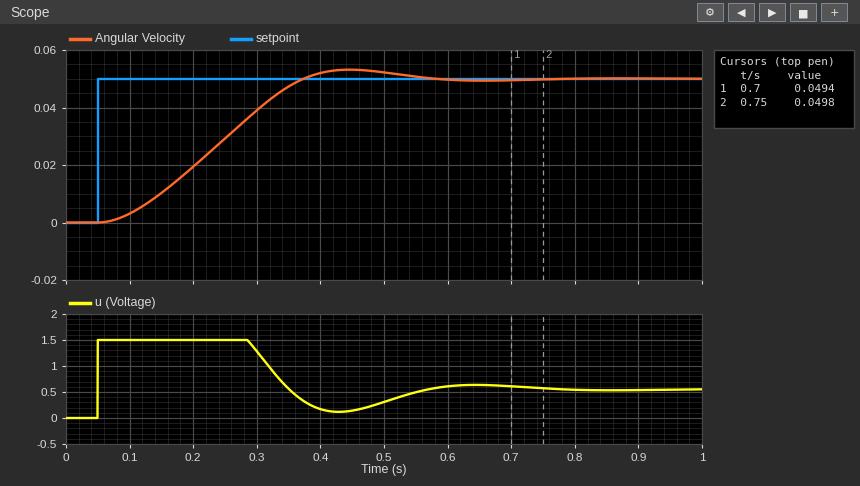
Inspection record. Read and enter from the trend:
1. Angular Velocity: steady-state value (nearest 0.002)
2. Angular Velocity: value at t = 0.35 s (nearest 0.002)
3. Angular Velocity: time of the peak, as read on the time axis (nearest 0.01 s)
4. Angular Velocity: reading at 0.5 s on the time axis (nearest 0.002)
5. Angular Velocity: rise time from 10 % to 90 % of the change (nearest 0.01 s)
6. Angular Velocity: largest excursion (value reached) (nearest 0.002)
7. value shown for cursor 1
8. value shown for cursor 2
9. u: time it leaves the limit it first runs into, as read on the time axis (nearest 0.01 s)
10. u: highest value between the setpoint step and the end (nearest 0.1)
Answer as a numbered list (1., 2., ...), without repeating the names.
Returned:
1. 0.050
2. 0.048
3. 0.45 s
4. 0.052
5. 0.22 s
6. 0.054
7. 0.0494
8. 0.0498
9. 0.29 s
10. 1.5
